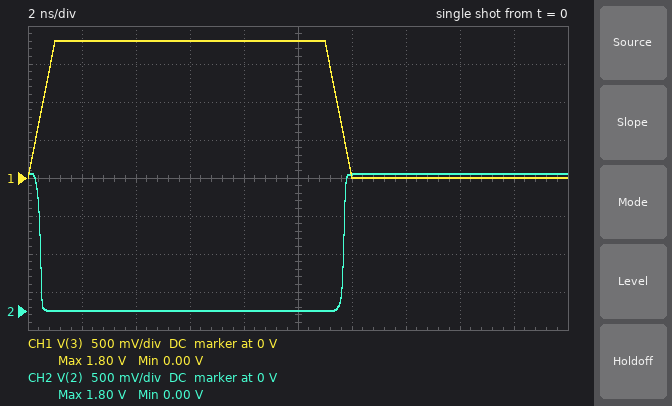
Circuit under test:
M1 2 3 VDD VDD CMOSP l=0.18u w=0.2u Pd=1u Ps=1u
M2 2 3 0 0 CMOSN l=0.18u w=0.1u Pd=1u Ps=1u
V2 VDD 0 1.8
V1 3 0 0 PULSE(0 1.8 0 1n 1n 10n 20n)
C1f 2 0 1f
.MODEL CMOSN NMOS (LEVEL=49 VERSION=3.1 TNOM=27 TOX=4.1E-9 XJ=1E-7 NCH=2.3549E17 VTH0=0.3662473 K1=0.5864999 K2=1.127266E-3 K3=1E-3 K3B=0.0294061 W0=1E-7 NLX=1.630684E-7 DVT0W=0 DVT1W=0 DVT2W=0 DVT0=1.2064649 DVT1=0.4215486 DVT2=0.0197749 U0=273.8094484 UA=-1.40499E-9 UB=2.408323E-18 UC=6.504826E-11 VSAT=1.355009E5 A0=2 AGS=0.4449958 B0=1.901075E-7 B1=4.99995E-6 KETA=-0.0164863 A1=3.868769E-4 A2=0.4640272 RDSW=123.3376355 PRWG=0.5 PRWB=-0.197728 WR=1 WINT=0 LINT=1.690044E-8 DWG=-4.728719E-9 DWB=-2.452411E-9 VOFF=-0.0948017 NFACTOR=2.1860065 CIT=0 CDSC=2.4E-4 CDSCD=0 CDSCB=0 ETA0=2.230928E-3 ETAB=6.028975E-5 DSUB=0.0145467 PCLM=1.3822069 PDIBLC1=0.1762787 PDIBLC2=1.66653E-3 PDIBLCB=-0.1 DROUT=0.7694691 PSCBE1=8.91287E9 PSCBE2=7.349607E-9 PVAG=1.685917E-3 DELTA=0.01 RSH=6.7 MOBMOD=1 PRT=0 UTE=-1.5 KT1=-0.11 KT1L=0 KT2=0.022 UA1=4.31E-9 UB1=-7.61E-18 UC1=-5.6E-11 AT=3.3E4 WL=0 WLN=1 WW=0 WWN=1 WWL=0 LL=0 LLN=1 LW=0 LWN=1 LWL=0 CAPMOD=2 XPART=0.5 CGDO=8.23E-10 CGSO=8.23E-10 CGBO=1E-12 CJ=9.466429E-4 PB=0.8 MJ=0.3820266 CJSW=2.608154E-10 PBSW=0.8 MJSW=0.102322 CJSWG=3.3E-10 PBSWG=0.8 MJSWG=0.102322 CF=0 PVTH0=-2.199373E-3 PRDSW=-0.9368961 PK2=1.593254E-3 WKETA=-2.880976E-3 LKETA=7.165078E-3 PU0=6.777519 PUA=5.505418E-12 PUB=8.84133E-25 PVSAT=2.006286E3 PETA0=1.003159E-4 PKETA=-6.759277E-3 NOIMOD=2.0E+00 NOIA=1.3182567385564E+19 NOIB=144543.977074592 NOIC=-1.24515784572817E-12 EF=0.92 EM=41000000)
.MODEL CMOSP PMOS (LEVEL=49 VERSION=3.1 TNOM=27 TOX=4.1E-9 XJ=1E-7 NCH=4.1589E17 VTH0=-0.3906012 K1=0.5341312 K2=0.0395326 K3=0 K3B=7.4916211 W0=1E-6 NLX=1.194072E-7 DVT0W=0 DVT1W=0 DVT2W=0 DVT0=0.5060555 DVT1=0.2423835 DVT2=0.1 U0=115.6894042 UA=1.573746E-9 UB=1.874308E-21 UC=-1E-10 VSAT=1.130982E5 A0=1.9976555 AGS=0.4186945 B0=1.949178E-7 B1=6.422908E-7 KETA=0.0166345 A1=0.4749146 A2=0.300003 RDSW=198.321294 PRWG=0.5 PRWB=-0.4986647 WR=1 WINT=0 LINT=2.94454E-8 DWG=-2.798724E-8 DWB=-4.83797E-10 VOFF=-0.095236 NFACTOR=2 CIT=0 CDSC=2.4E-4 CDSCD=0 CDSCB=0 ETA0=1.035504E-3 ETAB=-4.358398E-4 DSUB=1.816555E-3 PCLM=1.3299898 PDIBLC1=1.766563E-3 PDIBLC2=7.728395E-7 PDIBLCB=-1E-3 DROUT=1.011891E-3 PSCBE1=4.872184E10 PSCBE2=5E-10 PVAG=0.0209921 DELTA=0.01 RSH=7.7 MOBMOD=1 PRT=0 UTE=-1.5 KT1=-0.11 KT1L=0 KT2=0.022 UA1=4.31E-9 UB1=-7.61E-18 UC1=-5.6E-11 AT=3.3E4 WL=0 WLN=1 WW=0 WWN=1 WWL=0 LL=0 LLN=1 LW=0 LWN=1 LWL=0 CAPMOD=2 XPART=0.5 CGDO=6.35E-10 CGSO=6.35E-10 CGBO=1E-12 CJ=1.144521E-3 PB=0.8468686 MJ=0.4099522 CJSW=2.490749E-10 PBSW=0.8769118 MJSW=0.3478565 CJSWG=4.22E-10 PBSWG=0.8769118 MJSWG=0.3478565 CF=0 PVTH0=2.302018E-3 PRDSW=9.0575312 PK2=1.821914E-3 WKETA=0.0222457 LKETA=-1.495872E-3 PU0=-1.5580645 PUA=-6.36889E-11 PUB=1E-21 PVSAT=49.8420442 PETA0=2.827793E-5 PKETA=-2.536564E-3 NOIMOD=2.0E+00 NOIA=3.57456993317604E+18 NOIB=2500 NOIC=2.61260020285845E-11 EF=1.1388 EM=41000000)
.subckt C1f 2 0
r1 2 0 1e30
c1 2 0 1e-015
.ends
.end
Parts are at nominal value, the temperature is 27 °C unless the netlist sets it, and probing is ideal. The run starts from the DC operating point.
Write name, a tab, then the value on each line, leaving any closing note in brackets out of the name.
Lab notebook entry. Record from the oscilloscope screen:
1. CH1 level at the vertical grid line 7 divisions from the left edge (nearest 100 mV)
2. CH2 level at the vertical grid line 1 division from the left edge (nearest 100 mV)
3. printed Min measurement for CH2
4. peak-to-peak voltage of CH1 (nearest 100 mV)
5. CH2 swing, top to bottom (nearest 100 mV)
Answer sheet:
CH1 level at the vertical grid line 7 divisions from the left edge	0 V
CH2 level at the vertical grid line 1 division from the left edge	0 V
printed Min measurement for CH2	0.00 V
peak-to-peak voltage of CH1	1.8 V
CH2 swing, top to bottom	1.8 V
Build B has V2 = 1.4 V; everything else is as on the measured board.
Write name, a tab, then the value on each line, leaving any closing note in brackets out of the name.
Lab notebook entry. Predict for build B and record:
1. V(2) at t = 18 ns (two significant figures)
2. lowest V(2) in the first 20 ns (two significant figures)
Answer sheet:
V(2) at t = 18 ns	1.4 V
lowest V(2) in the first 20 ns	-1.9 mV
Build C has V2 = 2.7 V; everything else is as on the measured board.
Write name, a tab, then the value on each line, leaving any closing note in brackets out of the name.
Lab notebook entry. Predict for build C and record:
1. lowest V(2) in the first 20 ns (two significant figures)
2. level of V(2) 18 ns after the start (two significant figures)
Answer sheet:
lowest V(2) in the first 20 ns	37 mV
level of V(2) 18 ns after the start	2.7 V
